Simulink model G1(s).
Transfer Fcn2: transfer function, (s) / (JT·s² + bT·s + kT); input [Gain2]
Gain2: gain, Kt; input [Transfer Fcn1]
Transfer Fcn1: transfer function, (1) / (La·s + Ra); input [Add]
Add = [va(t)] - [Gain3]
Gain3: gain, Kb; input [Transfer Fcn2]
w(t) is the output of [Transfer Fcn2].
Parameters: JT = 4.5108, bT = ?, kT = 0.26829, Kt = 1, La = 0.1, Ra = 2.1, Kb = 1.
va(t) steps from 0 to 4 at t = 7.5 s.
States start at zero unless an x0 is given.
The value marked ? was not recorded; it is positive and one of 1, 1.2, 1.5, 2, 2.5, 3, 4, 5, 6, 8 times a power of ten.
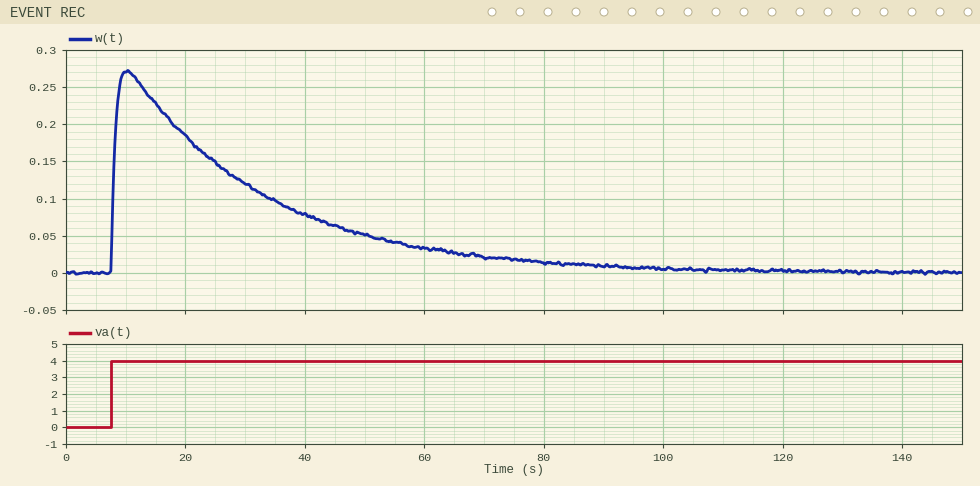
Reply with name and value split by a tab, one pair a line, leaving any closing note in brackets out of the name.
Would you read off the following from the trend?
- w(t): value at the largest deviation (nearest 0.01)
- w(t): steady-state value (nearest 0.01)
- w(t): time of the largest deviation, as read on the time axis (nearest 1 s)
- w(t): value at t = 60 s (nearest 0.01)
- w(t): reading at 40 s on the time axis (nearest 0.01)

w(t): value at the largest deviation	0.27
w(t): steady-state value	0.00
w(t): time of the largest deviation, as read on the time axis	10 s
w(t): value at t = 60 s	0.03
w(t): reading at 40 s on the time axis	0.08
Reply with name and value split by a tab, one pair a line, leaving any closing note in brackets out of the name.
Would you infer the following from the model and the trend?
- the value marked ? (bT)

the value marked ?	6
